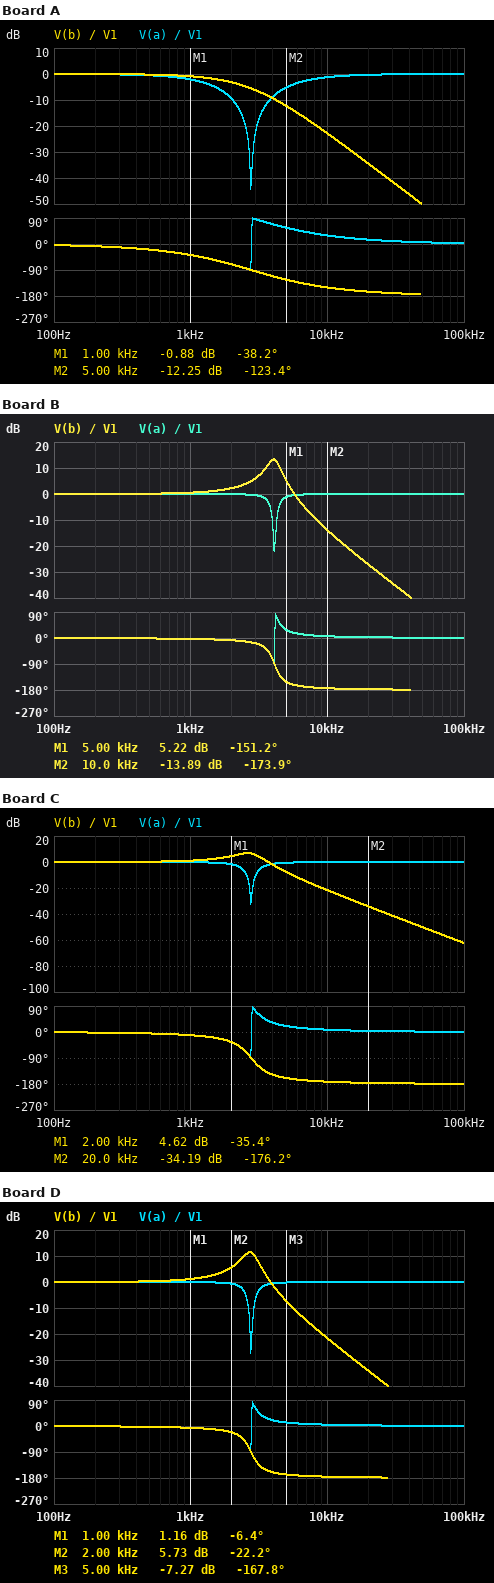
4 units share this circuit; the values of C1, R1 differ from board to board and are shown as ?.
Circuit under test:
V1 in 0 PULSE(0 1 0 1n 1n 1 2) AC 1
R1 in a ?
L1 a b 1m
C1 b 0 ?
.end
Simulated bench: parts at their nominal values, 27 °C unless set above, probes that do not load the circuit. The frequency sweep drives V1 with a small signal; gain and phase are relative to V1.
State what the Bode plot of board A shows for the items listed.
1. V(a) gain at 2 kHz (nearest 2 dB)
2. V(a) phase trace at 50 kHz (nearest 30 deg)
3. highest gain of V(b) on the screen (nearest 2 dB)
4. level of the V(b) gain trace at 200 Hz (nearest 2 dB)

-10 dB
0 deg
0 dB
0 dB
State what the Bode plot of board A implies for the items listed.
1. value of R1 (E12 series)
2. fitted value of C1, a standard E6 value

33 Ω
3.3 µF
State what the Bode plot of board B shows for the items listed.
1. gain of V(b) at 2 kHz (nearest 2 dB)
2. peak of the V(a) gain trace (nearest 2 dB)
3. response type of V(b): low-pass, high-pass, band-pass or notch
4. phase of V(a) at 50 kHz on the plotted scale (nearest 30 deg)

2 dB
0 dB
low-pass
0 deg
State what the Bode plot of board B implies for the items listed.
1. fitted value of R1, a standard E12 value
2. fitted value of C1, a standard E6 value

5.6 Ω
1.5 µF
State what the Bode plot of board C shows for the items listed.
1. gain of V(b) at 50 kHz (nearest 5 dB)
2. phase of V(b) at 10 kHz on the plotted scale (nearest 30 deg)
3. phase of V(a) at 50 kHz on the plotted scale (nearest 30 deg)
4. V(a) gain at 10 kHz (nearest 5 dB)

-50 dB
-180 deg
0 deg
0 dB
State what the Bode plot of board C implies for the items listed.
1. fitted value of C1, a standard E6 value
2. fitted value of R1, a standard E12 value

3.3 µF
8.2 Ω
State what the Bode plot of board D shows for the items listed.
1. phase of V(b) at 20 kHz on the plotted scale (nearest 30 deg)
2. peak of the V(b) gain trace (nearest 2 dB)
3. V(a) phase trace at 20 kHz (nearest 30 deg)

-180 deg
12 dB
0 deg
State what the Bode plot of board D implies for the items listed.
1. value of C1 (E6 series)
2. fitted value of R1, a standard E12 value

3.3 µF
4.7 Ω
